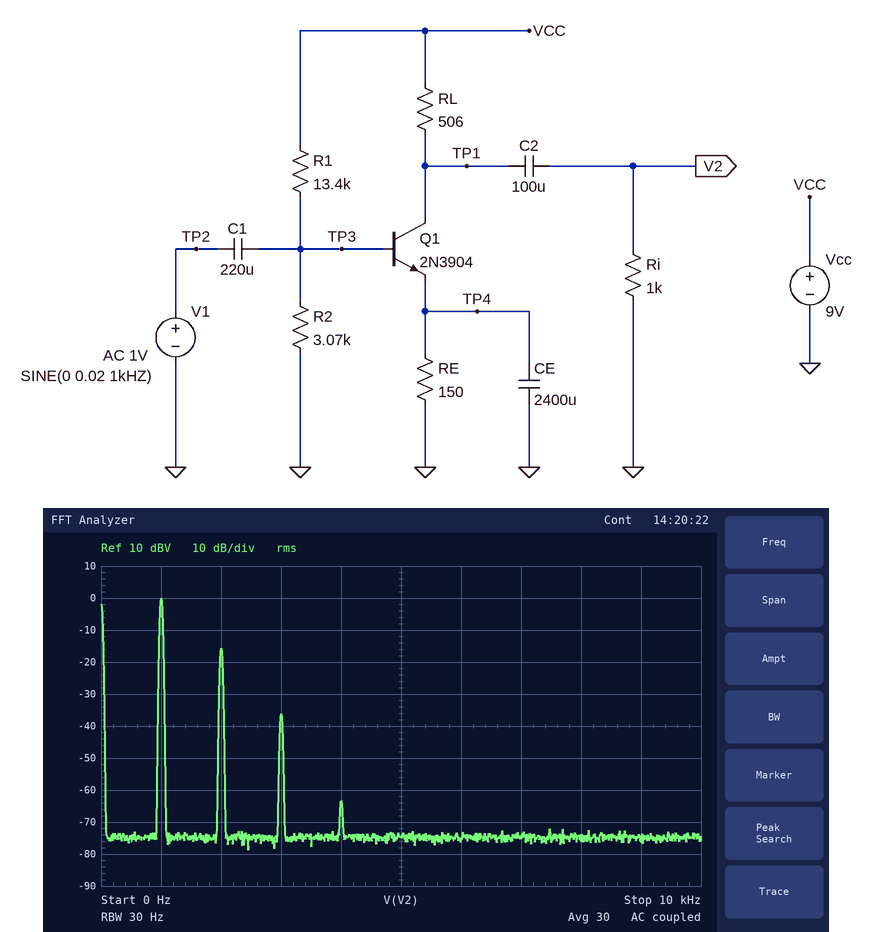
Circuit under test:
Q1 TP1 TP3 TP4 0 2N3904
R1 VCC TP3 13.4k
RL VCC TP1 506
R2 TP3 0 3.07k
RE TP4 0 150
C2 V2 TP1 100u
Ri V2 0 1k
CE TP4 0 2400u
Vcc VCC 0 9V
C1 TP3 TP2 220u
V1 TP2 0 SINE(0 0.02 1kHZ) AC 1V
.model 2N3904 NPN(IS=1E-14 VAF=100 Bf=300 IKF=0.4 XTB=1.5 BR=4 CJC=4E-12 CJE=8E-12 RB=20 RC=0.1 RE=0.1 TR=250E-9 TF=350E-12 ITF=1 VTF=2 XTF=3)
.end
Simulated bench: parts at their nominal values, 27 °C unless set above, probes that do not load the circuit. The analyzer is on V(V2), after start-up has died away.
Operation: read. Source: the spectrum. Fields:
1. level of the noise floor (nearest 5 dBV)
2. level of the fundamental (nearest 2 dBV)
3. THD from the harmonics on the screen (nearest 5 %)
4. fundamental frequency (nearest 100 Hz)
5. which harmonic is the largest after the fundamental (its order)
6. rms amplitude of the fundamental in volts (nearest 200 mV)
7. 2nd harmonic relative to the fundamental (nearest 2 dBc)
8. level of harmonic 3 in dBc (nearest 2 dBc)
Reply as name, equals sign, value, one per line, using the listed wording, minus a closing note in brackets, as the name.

level of the noise floor = -75 dBV
level of the fundamental = 0 dBV
THD from the harmonics on the screen = 15 %
fundamental frequency = 1.0 kHz
which harmonic is the largest after the fundamental = 2
rms amplitude of the fundamental in volts = 1.0 V
2nd harmonic relative to the fundamental = -16 dBc
level of harmonic 3 in dBc = -36 dBc
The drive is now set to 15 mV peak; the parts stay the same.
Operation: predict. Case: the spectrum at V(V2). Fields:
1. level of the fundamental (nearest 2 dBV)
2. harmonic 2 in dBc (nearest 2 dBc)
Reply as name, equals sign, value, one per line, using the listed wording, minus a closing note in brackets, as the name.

level of the fundamental = -2 dBV
harmonic 2 in dBc = -18 dBc
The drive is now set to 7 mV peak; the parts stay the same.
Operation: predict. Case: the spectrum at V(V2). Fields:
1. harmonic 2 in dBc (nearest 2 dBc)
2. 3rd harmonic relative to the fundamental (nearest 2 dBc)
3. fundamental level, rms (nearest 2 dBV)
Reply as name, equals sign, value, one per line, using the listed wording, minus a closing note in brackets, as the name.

harmonic 2 in dBc = -24 dBc
3rd harmonic relative to the fundamental = -54 dBc
fundamental level, rms = -8 dBV
